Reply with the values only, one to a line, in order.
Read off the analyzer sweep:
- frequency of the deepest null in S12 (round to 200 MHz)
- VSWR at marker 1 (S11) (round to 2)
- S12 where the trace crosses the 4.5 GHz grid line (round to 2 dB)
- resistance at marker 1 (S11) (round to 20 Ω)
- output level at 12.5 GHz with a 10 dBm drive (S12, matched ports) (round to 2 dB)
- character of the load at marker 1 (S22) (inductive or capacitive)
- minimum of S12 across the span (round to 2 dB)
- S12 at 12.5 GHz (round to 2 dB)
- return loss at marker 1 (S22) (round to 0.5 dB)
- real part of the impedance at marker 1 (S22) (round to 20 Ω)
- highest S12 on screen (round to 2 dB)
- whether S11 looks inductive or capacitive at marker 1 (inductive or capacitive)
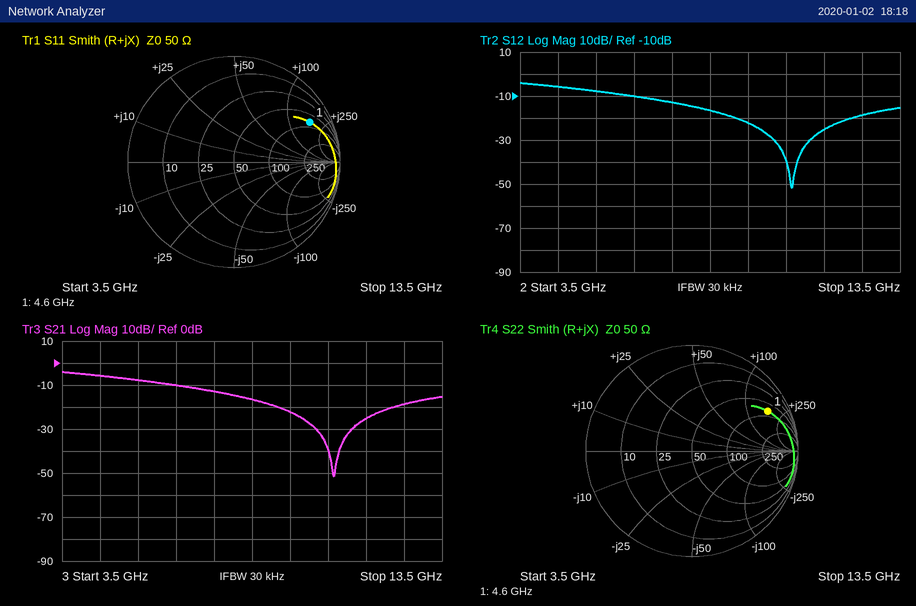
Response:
10.6 GHz
10
-6 dB
80 Ω
-8 dBm
inductive
-52 dB
-18 dB
2.0 dB
80 Ω
-4 dB
inductive
